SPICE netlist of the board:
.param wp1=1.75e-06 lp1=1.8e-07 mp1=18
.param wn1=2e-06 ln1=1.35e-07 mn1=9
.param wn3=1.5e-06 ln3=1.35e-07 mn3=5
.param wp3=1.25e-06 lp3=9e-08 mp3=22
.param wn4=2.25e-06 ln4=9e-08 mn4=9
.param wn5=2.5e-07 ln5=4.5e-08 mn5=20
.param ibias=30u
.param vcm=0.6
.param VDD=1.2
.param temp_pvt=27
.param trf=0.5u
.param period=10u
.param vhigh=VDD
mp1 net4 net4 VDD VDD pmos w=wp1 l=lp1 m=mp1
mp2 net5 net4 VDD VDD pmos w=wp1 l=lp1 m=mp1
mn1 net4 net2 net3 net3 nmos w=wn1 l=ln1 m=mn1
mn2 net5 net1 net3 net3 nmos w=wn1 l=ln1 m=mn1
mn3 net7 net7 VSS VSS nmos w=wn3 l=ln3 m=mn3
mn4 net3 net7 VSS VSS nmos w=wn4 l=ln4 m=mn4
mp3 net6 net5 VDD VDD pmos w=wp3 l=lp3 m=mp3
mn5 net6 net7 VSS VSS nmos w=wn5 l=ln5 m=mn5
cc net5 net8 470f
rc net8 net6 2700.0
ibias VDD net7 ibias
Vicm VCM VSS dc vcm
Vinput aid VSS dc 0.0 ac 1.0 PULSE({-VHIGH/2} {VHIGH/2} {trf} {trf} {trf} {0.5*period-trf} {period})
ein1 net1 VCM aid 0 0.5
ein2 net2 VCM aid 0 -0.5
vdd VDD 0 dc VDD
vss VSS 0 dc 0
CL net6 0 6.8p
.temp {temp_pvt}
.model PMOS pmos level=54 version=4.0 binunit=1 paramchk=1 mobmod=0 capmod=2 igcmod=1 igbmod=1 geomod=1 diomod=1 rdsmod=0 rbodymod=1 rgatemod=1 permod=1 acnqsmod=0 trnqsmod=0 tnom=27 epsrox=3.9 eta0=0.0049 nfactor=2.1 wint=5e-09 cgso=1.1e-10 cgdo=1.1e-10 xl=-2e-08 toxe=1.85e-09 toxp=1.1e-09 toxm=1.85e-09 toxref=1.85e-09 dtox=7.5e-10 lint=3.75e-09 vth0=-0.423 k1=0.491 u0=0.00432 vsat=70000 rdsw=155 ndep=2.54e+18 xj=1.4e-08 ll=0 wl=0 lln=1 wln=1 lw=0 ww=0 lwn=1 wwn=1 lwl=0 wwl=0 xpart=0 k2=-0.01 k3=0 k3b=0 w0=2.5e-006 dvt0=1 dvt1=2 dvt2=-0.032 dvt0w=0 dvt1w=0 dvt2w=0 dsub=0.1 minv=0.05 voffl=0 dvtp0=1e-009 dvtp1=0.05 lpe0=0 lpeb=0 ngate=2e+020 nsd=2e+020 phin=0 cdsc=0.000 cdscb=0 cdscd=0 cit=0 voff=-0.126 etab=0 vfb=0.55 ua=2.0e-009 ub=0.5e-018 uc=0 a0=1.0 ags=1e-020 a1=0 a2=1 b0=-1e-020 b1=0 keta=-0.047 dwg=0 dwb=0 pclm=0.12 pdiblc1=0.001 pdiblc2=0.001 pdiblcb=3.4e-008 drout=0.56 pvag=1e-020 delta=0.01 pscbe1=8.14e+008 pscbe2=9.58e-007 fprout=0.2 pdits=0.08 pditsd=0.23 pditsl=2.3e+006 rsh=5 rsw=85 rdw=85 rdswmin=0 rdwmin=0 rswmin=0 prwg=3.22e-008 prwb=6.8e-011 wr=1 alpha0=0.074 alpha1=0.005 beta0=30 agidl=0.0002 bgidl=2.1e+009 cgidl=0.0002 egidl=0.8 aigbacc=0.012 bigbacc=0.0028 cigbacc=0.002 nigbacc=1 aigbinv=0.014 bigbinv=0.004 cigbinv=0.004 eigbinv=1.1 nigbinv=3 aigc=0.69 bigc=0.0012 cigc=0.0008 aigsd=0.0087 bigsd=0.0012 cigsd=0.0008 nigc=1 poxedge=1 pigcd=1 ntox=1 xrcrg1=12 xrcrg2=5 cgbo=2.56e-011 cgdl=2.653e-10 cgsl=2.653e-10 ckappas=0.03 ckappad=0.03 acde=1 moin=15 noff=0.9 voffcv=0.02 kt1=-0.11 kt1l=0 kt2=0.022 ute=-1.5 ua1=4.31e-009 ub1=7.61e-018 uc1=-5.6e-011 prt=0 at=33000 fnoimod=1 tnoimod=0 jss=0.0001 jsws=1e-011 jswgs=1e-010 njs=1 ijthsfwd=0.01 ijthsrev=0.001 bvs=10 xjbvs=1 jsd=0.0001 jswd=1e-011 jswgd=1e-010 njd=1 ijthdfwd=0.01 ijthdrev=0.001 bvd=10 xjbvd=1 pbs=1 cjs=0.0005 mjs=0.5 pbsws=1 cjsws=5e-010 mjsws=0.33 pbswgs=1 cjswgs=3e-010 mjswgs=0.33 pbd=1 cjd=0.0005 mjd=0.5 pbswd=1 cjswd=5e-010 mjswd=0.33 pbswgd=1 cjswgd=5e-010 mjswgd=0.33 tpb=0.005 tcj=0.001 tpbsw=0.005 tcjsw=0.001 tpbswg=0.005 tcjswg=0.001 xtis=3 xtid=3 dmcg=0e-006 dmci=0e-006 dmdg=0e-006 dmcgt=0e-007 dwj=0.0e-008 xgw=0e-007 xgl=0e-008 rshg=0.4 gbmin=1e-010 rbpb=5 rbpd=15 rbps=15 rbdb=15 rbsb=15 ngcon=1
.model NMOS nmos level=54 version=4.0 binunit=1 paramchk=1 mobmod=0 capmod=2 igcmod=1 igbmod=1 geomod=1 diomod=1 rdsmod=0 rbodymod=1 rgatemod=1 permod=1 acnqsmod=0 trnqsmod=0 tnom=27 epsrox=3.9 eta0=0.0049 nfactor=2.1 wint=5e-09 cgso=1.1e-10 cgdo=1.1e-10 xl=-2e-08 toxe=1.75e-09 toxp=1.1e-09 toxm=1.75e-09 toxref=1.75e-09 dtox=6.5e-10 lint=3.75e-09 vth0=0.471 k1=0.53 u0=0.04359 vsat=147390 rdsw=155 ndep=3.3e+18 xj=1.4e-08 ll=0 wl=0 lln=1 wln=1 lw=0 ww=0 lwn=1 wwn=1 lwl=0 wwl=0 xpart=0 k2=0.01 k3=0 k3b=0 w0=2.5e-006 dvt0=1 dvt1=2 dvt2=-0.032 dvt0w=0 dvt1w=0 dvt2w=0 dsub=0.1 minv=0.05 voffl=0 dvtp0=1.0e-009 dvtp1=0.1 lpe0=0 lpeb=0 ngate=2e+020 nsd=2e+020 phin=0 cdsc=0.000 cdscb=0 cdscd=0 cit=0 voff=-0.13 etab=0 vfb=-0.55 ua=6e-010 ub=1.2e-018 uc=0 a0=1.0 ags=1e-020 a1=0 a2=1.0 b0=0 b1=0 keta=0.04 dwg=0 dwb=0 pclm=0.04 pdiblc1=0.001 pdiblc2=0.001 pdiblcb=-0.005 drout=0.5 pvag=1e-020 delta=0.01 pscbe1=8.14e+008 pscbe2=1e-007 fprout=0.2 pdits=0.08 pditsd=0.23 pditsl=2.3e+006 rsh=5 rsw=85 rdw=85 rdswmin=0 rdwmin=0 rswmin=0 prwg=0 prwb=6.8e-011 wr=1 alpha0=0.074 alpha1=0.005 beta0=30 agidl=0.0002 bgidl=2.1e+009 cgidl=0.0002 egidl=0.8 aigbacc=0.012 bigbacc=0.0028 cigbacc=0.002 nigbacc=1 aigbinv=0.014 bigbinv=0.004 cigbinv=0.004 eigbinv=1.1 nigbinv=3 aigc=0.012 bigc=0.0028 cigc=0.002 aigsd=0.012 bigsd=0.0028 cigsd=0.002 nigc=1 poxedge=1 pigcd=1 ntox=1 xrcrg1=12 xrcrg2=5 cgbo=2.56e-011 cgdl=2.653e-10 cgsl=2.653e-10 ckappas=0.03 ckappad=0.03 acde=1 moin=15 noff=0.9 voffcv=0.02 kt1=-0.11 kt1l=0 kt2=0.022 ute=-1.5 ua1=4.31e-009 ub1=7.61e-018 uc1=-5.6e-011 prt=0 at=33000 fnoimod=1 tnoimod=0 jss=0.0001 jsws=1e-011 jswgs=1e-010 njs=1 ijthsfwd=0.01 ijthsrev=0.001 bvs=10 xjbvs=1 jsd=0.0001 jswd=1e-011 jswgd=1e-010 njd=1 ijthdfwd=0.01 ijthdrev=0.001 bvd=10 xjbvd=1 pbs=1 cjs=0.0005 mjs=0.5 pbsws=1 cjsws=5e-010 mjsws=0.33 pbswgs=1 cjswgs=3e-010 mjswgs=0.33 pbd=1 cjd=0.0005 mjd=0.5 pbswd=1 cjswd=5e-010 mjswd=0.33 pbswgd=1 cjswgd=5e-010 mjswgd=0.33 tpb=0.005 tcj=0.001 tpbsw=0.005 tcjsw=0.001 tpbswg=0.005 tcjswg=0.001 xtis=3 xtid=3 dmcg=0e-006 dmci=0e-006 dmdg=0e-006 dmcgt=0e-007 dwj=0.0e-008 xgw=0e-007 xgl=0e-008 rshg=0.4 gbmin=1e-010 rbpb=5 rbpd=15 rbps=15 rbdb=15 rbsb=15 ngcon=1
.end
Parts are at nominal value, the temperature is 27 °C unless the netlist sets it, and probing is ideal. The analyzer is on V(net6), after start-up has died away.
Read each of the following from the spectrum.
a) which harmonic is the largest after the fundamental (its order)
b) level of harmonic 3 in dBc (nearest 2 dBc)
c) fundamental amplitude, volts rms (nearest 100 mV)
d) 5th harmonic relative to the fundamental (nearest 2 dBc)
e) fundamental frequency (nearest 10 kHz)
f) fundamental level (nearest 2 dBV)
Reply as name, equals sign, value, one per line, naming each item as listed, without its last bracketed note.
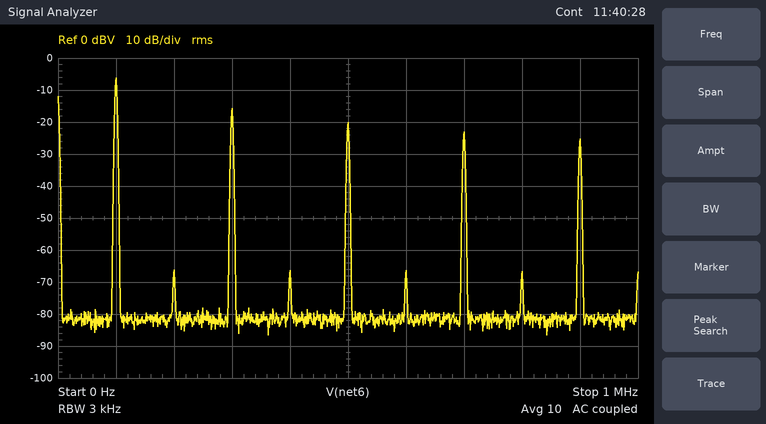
which harmonic is the largest after the fundamental = 3
level of harmonic 3 in dBc = -10 dBc
fundamental amplitude, volts rms = 500 mV
5th harmonic relative to the fundamental = -14 dBc
fundamental frequency = 100 kHz
fundamental level = -6 dBV
